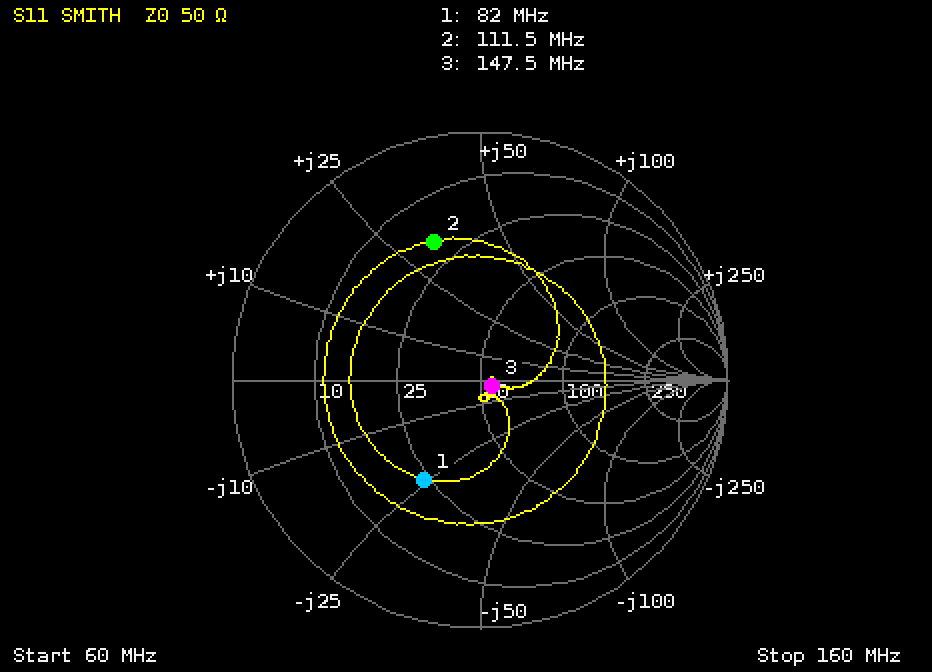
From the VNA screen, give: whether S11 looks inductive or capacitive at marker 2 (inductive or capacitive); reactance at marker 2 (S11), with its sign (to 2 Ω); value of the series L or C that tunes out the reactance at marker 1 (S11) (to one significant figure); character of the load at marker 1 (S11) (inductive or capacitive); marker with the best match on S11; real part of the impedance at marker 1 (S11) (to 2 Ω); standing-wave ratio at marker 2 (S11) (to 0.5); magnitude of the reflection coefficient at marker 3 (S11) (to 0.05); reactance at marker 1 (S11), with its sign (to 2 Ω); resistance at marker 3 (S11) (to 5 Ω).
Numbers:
inductive
+32 Ω
50 nH
capacitive
marker 3
24 Ω
4.0
0.05
-24 Ω
55 Ω
